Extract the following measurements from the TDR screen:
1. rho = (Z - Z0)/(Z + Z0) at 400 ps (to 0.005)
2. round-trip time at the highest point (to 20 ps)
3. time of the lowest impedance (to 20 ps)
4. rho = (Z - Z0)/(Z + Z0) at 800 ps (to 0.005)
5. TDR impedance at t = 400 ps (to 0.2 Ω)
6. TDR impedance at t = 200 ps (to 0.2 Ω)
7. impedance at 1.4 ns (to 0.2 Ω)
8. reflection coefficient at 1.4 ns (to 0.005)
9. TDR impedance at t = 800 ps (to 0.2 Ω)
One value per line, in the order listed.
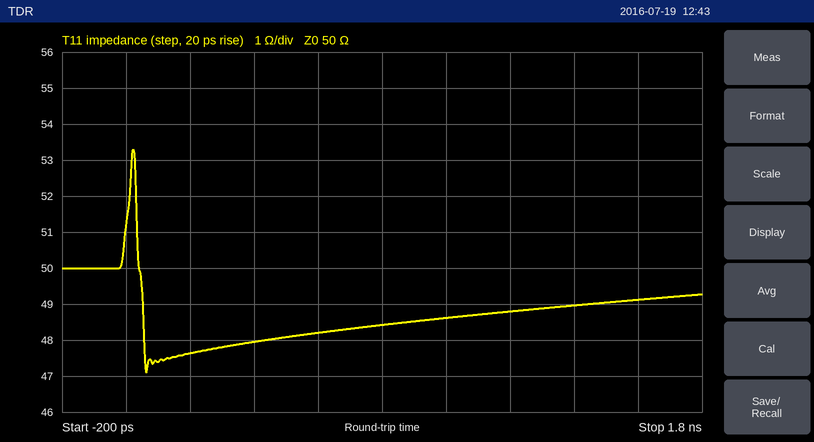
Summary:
-0.020
20 ps
60 ps
-0.015
48.0 Ω
47.6 Ω
49.0 Ω
-0.010
48.4 Ω
